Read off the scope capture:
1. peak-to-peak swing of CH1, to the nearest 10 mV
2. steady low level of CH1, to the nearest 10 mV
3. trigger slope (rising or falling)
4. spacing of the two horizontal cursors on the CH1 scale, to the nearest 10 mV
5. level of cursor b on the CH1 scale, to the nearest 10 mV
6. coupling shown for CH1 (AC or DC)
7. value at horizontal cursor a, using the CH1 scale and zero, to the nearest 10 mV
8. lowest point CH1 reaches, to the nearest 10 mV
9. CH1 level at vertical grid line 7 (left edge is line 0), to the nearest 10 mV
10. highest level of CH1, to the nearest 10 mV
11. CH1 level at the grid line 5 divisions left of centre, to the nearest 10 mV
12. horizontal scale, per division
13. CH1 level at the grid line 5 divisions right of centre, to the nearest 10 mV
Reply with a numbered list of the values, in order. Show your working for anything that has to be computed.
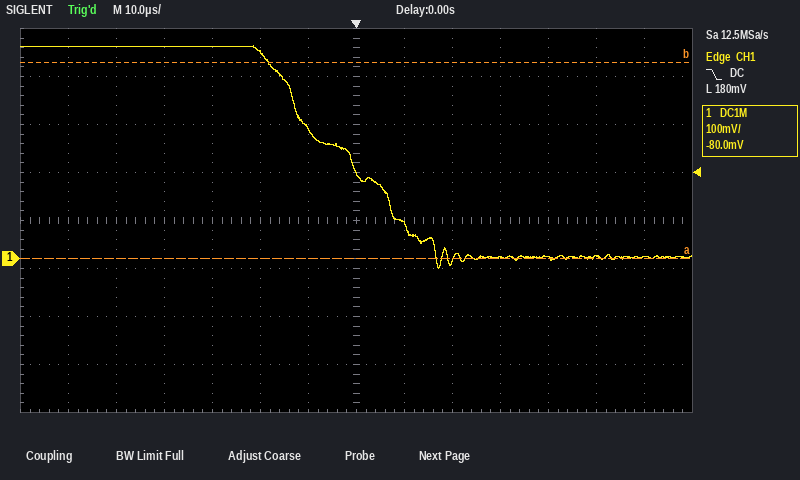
1. 440 mV − (-20 mV) = 460 mV
2. 0 mV
3. falling
4. 410 mV
5. 410 mV
6. DC
7. 0 mV
8. -20 mV
9. 180 mV
10. 440 mV
11. 440 mV
12. 10 µs
13. 10 mV
